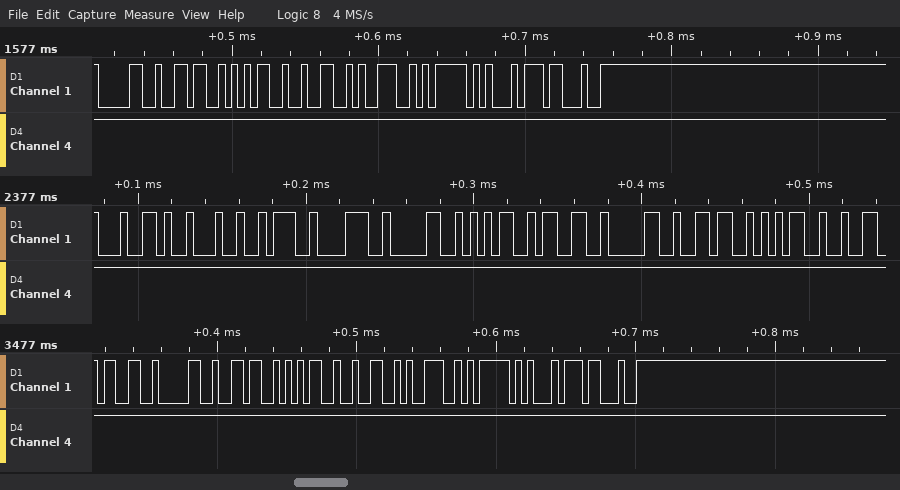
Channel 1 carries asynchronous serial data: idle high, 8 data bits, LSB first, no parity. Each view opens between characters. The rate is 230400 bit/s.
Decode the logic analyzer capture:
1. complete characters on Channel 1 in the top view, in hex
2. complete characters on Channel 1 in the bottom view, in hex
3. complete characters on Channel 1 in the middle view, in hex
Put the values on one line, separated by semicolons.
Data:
30, 36, 35, 32, 39, 7D, D1, 23; 33, 30, 36, 35, 32, 39, 7D, D1, 23; 64, 22, 3A, 38, 30, 35, 33, 30, 36, 35
